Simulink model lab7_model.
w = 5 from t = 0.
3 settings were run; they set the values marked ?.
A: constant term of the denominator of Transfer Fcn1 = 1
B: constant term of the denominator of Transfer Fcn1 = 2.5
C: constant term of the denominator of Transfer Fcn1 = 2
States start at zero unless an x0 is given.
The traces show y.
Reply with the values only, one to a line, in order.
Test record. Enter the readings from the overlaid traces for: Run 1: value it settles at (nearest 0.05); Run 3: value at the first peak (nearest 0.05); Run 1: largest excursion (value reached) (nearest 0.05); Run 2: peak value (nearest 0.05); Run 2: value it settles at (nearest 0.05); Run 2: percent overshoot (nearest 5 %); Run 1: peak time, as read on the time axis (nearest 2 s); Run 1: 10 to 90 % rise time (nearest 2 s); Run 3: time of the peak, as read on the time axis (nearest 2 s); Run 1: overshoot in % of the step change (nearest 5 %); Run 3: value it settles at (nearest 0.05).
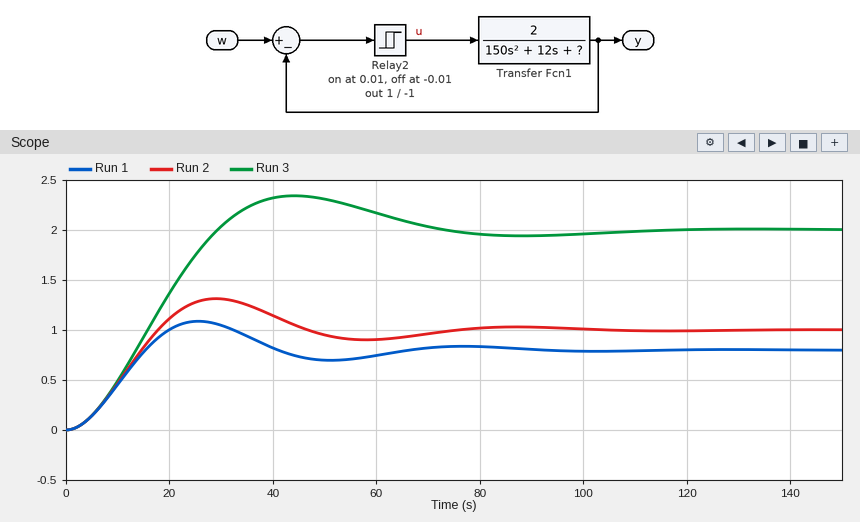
0.80
2.35
1.10
1.30
1.00
30 %
26 s
10 s
44 s
35 %
2.00
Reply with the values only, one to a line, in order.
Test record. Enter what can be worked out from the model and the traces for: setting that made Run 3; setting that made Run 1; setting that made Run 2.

A
B
C
